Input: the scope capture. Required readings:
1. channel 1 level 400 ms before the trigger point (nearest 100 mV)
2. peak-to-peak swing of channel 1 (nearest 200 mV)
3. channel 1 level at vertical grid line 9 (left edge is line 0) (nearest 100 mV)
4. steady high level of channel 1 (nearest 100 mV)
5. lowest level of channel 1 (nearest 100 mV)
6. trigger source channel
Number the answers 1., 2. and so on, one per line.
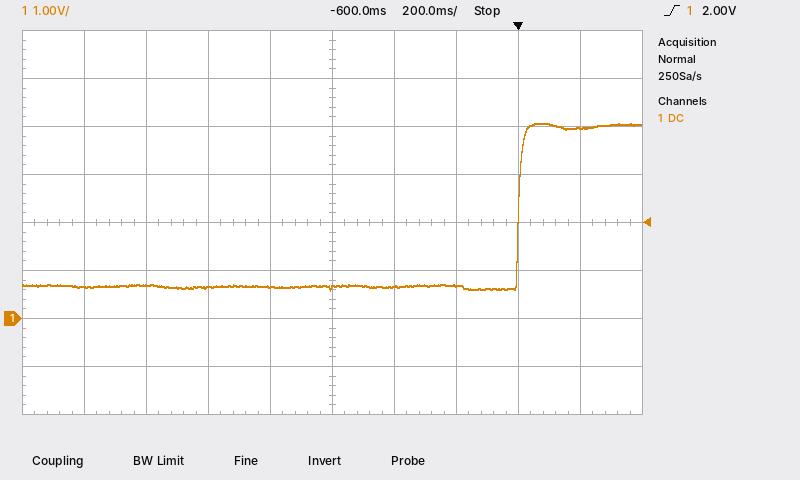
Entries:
1. 700 mV
2. 3.4 V
3. 4.0 V
4. 4.0 V
5. 600 mV
6. channel 1
